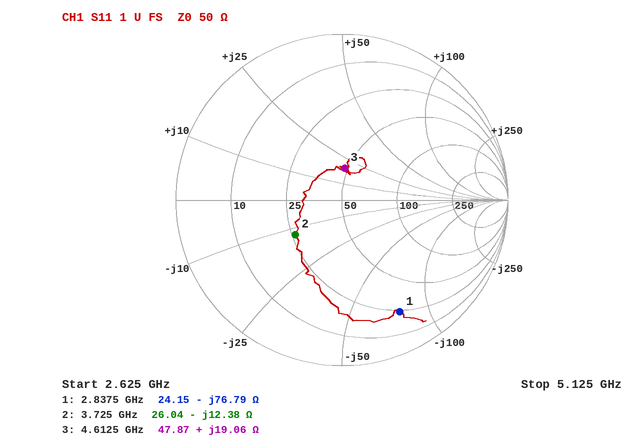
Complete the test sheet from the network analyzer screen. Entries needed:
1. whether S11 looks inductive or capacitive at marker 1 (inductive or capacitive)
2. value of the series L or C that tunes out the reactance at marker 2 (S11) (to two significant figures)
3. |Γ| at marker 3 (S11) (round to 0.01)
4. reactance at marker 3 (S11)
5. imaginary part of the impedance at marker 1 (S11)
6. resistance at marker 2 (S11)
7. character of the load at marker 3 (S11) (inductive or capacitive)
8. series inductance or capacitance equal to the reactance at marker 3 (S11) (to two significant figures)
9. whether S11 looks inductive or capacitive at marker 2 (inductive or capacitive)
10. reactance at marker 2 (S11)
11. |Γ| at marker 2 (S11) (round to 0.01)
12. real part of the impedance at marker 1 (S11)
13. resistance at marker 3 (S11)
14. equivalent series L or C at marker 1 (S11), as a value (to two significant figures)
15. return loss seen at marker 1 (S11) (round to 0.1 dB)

capacitive
530 pH
0.19
+19.06 Ω
-76.79 Ω
26.04 Ω
inductive
660 pH
capacitive
-12.38 Ω
0.35
24.15 Ω
47.87 Ω
730 fF
2.4 dB
